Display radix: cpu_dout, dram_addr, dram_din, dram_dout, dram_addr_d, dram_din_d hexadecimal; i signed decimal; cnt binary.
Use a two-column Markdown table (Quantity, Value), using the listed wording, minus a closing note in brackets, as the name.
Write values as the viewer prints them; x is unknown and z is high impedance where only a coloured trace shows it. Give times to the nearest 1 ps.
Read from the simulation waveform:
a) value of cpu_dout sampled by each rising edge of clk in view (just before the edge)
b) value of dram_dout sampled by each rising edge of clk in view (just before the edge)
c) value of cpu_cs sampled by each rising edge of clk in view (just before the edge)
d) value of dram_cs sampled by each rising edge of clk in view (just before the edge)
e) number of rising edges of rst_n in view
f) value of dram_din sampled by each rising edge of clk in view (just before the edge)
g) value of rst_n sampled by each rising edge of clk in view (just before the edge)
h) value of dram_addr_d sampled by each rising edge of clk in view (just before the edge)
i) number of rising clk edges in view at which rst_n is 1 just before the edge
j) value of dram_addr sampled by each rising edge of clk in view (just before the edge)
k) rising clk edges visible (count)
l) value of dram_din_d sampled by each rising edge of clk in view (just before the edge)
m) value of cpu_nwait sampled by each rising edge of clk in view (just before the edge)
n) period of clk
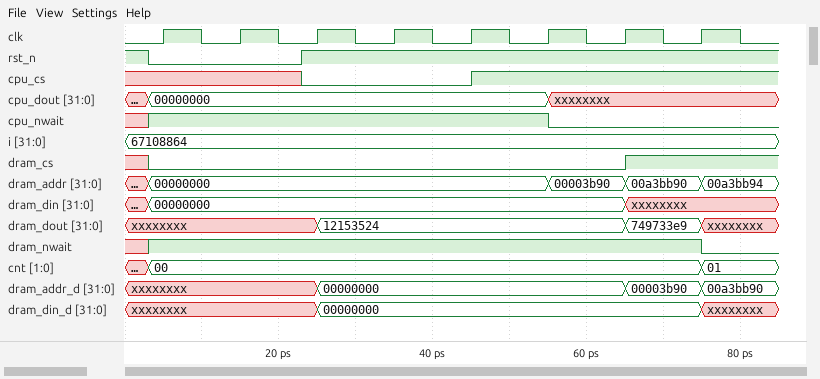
| Quantity | Value |
|---|---|
| value of cpu_dout sampled by each rising edge of clk in view | 00000000, 00000000, 00000000, 00000000, 00000000, 00000000, xxxxxxxx, xxxxxxxx |
| value of dram_dout sampled by each rising edge of clk in view | xxxxxxxx, xxxxxxxx, xxxxxxxx, 12153524, 12153524, 12153524, 12153524, 749733e9 |
| value of cpu_cs sampled by each rising edge of clk in view | x x 0 0 0 1 1 1 |
| value of dram_cs sampled by each rising edge of clk in view | 0 0 0 0 0 0 0 1 |
| number of rising edges of rst_n in view | 1 |
| value of dram_din sampled by each rising edge of clk in view | 00000000, 00000000, 00000000, 00000000, 00000000, 00000000, 00000000, xxxxxxxx |
| value of rst_n sampled by each rising edge of clk in view | 0 0 1 1 1 1 1 1 |
| value of dram_addr_d sampled by each rising edge of clk in view | xxxxxxxx, xxxxxxxx, xxxxxxxx, 00000000, 00000000, 00000000, 00000000, 00003b90 |
| number of rising clk edges in view at which rst_n is 1 just before the edge | 6 |
| value of dram_addr sampled by each rising edge of clk in view | 00000000, 00000000, 00000000, 00000000, 00000000, 00000000, 00003b90, 00a3bb90 |
| rising clk edges visible | 8 |
| value of dram_din_d sampled by each rising edge of clk in view | xxxxxxxx, xxxxxxxx, xxxxxxxx, 00000000, 00000000, 00000000, 00000000, 00000000 |
| value of cpu_nwait sampled by each rising edge of clk in view | 1 1 1 1 1 1 0 0 |
| period of clk | 10 ps |
